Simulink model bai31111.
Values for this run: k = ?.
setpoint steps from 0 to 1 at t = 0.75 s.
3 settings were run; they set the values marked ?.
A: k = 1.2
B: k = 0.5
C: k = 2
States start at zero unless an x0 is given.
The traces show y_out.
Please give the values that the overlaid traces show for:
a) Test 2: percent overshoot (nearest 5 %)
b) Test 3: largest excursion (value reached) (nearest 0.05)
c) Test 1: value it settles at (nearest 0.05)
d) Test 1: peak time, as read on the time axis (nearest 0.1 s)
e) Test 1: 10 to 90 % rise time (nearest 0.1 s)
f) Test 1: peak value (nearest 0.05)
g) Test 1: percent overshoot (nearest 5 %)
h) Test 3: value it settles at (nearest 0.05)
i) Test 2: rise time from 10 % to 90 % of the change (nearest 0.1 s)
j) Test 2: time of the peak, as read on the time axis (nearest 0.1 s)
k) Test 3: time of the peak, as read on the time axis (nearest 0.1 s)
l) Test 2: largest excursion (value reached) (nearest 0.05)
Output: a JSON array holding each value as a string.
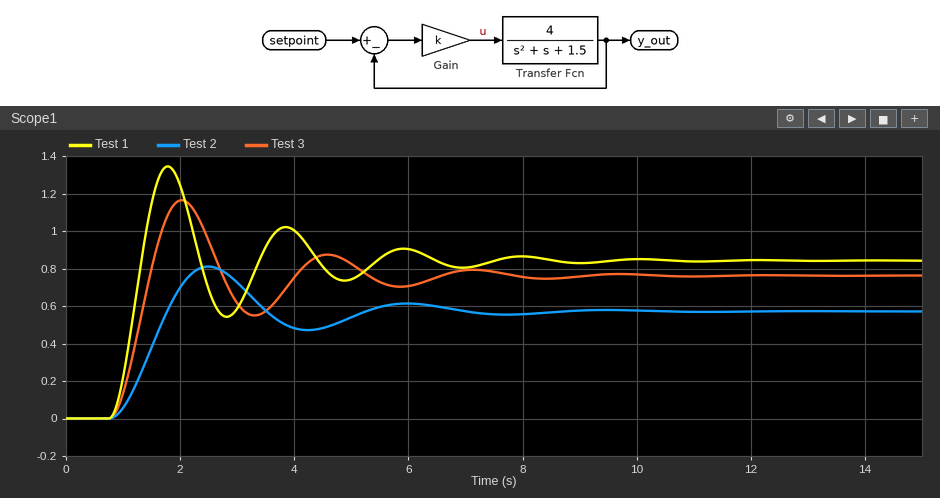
["40 %", "1.15", "0.85", "1.8 s", "0.4 s", "1.35", "60 %", "0.75", "0.7 s", "2.5 s", "2.0 s", "0.80"]
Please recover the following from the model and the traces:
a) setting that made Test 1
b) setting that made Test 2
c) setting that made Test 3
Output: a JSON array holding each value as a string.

["C", "B", "A"]
